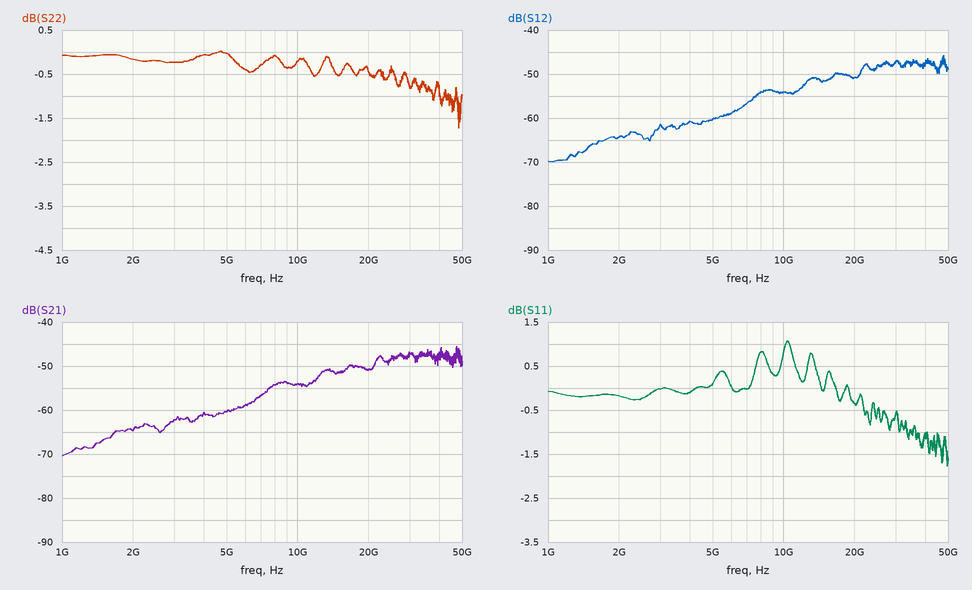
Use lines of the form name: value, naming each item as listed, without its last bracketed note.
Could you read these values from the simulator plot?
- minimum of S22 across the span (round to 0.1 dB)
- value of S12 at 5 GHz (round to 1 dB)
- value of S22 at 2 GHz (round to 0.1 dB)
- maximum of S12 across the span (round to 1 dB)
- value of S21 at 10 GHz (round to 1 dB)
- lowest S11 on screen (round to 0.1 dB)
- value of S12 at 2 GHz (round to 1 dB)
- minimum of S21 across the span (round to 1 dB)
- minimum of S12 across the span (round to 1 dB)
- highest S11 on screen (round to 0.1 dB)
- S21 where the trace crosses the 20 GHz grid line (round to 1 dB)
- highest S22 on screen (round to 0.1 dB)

minimum of S22 across the span: -1.7 dB
value of S12 at 5 GHz: -60 dB
value of S22 at 2 GHz: -0.2 dB
maximum of S12 across the span: -46 dB
value of S21 at 10 GHz: -54 dB
lowest S11 on screen: -1.8 dB
value of S12 at 2 GHz: -64 dB
minimum of S21 across the span: -70 dB
minimum of S12 across the span: -70 dB
highest S11 on screen: 1.1 dB
S21 where the trace crosses the 20 GHz grid line: -51 dB
highest S22 on screen: 0.0 dB
